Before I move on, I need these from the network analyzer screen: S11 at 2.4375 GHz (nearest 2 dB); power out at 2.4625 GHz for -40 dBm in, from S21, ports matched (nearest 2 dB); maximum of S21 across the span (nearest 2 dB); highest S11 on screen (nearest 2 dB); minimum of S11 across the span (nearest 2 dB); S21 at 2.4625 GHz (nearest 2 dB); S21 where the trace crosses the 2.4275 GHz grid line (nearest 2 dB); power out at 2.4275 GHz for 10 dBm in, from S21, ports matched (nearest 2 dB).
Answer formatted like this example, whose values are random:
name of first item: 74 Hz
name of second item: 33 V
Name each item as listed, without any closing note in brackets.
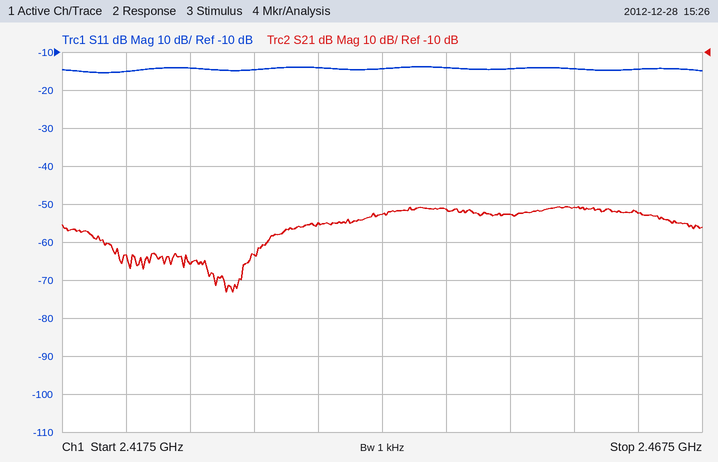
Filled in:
S11 at 2.4375 GHz: -14 dB
power out at 2.4625 GHz for -40 dBm in, from S21, ports matched: -92 dBm
maximum of S21 across the span: -50 dB
highest S11 on screen: -14 dB
minimum of S11 across the span: -16 dB
S21 at 2.4625 GHz: -52 dB
S21 where the trace crosses the 2.4275 GHz grid line: -66 dB
power out at 2.4275 GHz for 10 dBm in, from S21, ports matched: -56 dBm
